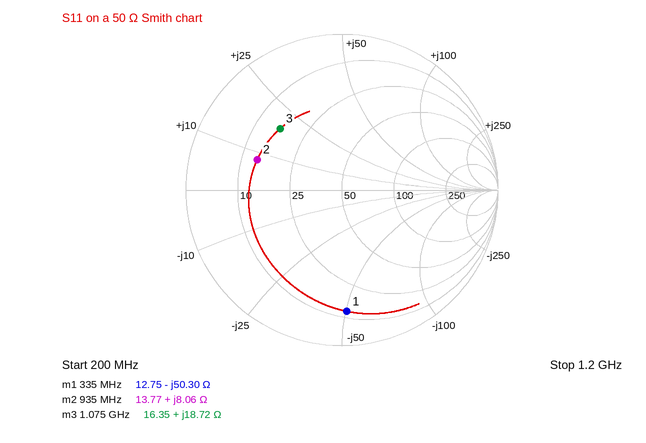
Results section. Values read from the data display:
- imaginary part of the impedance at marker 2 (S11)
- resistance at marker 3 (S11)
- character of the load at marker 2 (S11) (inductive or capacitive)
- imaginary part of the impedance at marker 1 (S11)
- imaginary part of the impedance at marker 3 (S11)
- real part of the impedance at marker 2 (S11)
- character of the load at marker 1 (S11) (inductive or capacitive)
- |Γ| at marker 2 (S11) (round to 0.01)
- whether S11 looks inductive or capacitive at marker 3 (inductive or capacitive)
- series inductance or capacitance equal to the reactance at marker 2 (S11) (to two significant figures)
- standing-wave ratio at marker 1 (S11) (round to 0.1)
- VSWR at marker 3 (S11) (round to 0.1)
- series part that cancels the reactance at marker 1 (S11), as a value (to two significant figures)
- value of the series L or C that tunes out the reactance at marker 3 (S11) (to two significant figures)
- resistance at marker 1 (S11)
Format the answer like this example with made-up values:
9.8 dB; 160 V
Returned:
+8.06 Ω; 16.35 Ω; inductive; -50.30 Ω; +18.72 Ω; 13.77 Ω; capacitive; 0.58; inductive; 1.4 nH; 8.0; 3.5; 24 nH; 7.9 pF; 12.75 Ω
